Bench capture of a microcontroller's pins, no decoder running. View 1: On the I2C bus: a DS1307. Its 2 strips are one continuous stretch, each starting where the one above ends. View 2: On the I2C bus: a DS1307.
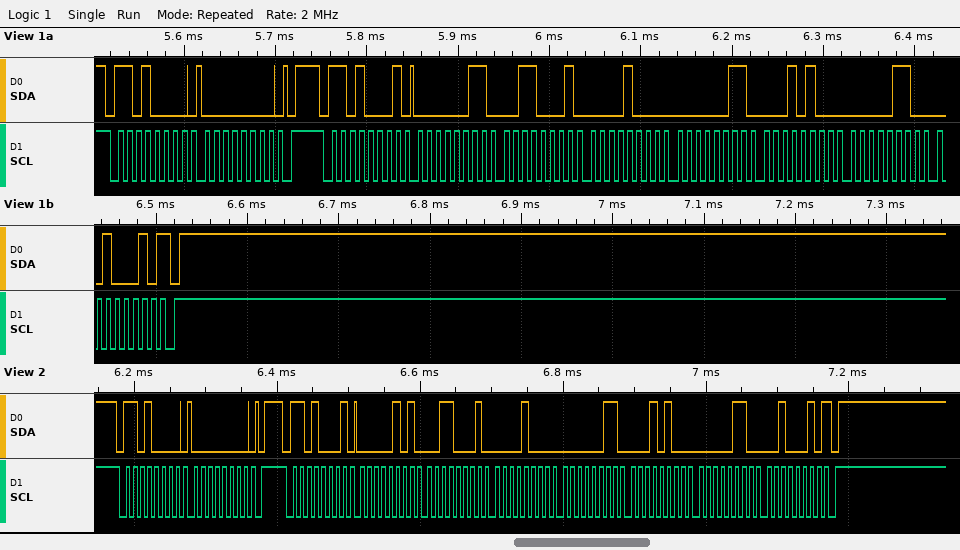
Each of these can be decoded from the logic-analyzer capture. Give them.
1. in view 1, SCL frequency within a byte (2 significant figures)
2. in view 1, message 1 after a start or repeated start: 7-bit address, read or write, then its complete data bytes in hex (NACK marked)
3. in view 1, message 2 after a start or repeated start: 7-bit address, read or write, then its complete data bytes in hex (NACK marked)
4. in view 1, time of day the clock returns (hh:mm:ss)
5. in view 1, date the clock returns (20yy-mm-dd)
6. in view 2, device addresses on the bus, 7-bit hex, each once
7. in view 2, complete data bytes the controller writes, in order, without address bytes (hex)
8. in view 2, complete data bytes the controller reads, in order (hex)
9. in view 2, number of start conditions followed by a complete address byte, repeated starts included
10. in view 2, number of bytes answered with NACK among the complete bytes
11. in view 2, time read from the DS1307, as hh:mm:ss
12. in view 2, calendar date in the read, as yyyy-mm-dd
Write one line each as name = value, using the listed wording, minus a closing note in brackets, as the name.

in view 1, SCL frequency within a byte = 100 kHz
in view 1, message 1 after a start or repeated start: 7-bit address, read or write, then its complete data bytes in hex = 0x68 write: 00
in view 1, message 2 after a start or repeated start: 7-bit address, read or write, then its complete data bytes in hex = 0x68 read: 03 31 08 03 14 06 22 NACK
in view 1, time of day the clock returns = 08:31:03
in view 1, date the clock returns = 2022-06-14
in view 2, device addresses on the bus, 7-bit hex, each once = 0x68
in view 2, complete data bytes the controller writes, in order, without address bytes = 00
in view 2, complete data bytes the controller reads, in order = 05 31 08 03 14 06 22
in view 2, number of start conditions followed by a complete address byte, repeated starts included = 2
in view 2, number of bytes answered with NACK among the complete bytes = 1
in view 2, time read from the DS1307, as hh:mm:ss = 08:31:05
in view 2, calendar date in the read, as yyyy-mm-dd = 2022-06-14
